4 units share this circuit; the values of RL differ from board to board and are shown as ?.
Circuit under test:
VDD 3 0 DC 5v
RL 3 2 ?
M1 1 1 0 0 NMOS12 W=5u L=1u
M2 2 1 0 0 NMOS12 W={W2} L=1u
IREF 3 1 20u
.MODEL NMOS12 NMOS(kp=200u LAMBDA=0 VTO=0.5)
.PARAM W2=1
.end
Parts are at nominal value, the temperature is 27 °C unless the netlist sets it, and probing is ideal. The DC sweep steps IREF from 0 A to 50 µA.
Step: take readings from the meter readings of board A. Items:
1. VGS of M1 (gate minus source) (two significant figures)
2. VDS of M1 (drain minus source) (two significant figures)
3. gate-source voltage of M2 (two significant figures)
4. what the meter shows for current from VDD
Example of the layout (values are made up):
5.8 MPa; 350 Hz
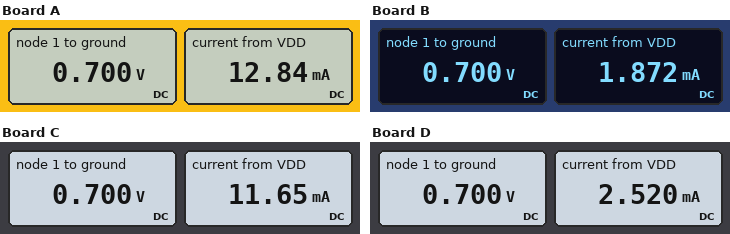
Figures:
700 mV; 700 mV; 700 mV; 12.84 mA
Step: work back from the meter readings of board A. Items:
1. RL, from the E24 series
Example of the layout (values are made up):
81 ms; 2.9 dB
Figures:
390 Ω
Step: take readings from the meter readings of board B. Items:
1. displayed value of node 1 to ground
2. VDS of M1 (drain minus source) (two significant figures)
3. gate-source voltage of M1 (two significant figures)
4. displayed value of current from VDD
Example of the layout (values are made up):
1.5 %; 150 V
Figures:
0.700 V; 700 mV; 700 mV; 1.872 mA
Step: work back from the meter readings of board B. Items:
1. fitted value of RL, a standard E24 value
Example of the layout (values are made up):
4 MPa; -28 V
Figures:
2.7 kΩ
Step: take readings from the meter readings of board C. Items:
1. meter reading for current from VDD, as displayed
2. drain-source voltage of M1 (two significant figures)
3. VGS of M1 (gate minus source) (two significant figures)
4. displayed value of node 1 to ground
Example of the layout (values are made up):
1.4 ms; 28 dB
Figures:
11.65 mA; 700 mV; 700 mV; 0.700 V
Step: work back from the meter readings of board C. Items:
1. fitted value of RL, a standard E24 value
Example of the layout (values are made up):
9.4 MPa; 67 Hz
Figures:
430 Ω
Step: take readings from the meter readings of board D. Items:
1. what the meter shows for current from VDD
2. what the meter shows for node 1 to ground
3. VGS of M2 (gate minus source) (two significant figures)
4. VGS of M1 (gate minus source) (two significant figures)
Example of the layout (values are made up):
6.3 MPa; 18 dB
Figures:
2.520 mA; 0.700 V; 700 mV; 700 mV
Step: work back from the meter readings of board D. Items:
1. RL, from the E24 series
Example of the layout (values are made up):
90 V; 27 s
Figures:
2 kΩ
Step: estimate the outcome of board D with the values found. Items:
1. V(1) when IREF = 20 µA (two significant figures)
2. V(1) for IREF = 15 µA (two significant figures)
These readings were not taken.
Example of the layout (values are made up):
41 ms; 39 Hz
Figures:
700 mV; 670 mV
